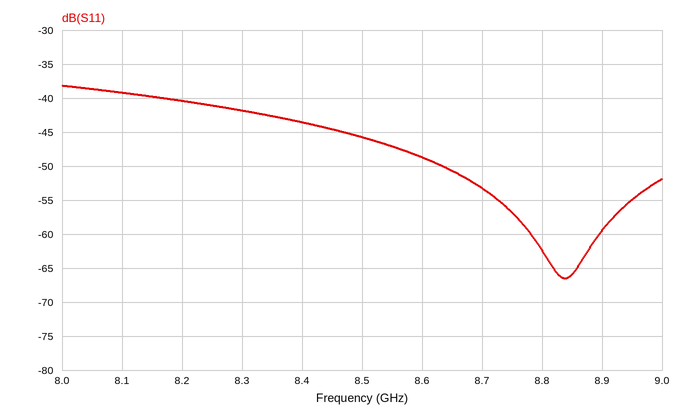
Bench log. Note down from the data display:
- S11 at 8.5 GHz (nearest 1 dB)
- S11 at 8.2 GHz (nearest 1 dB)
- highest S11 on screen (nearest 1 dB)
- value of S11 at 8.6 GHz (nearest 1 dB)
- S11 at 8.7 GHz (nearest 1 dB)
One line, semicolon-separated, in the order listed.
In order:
-46 dB; -40 dB; -38 dB; -49 dB; -53 dB
